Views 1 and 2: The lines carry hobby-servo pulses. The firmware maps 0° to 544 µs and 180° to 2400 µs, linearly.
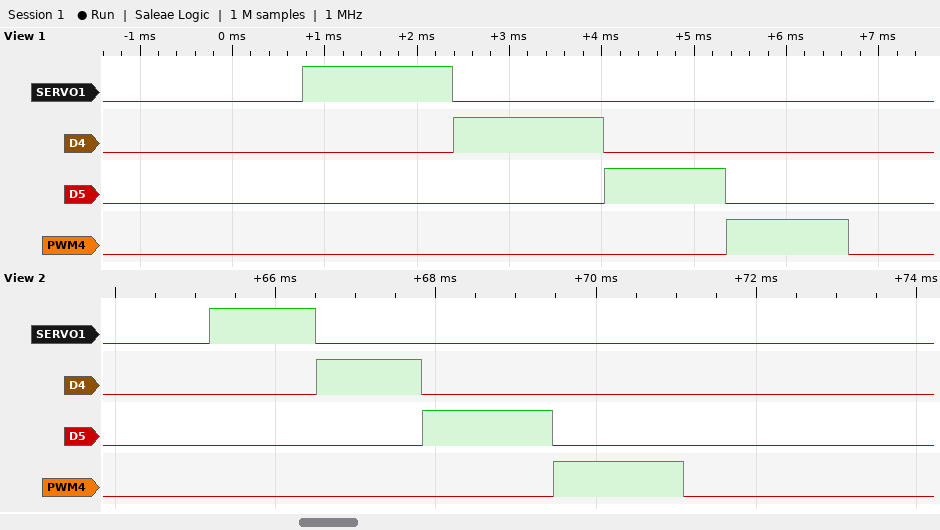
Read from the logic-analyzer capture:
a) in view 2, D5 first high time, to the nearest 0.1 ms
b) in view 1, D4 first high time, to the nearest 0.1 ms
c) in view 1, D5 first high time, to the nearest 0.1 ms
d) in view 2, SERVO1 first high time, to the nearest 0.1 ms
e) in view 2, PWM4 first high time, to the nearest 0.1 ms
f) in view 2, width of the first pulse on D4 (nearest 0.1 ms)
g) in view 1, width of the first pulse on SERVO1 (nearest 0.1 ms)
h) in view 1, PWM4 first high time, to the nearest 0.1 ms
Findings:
1.6 ms
1.6 ms
1.3 ms
1.3 ms
1.6 ms
1.3 ms
1.6 ms
1.3 ms
